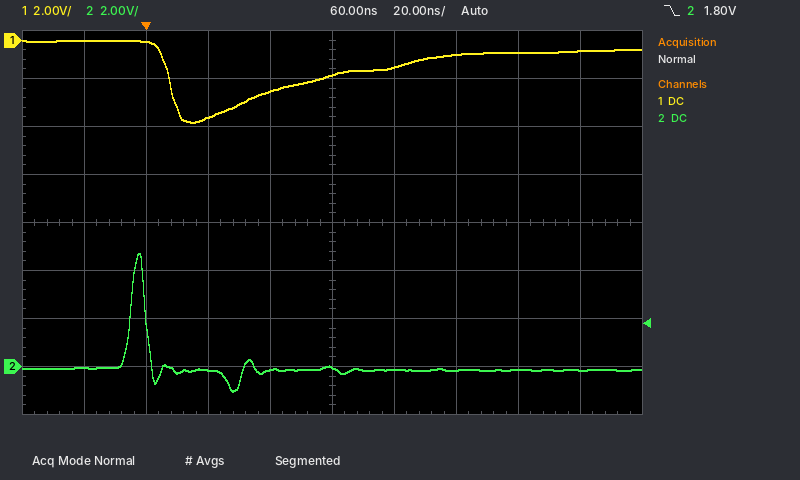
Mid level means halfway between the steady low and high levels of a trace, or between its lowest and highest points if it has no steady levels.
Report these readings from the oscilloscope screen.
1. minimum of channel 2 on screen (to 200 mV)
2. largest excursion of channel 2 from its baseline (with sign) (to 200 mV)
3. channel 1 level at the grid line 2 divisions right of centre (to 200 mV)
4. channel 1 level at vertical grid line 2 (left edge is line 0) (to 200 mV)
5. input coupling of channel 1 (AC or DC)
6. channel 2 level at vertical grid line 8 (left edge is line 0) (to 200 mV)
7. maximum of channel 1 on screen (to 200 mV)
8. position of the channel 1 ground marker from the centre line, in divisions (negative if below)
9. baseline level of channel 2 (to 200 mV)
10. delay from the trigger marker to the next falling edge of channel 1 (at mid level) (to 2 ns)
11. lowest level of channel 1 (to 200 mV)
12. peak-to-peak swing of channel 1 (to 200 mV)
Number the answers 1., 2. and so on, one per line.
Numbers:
1. -1.0 V
2. +4.8 V
3. -600 mV
4. 0.0 V
5. DC
6. -200 mV
7. 0.0 V
8. +3.8 div
9. -200 mV
10. 8 ns
11. -3.4 V
12. 3.4 V
